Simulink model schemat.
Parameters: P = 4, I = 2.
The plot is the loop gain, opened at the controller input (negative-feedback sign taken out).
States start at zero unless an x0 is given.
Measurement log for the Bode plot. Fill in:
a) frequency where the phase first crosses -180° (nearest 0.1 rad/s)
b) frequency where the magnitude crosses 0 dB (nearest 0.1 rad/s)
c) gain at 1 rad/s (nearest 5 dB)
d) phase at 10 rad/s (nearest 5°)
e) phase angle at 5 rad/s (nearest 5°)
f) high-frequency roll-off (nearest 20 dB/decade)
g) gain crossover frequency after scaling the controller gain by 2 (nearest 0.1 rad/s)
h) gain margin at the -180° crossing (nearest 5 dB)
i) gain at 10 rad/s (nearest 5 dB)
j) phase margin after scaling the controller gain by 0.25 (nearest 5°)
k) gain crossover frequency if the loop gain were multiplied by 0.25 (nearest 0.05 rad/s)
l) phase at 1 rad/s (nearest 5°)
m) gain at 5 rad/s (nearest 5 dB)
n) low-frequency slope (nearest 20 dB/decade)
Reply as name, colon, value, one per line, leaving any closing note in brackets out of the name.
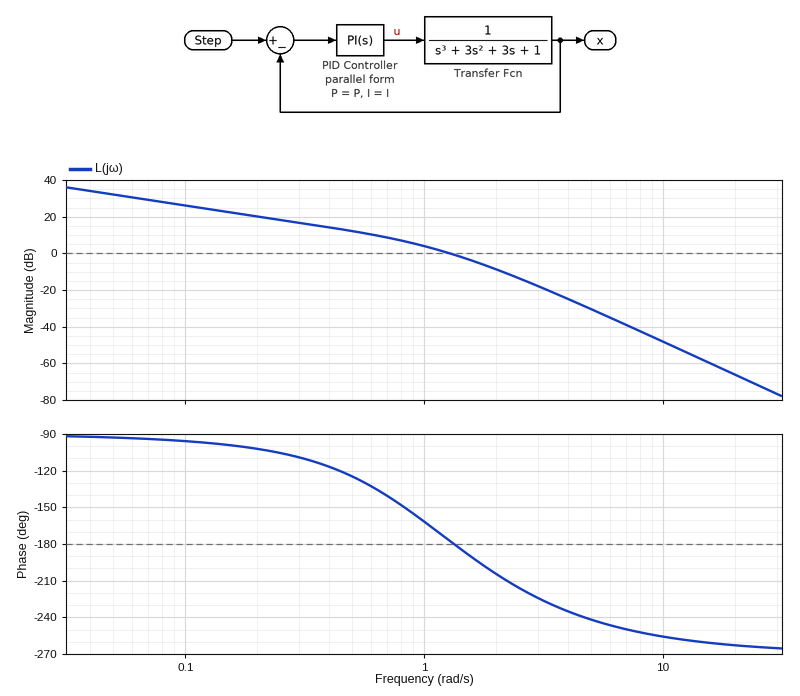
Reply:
frequency where the phase first crosses -180°: 1.3 rad/s
frequency where the magnitude crosses 0 dB: 1.3 rad/s
gain at 1 rad/s: 5 dB
phase at 10 rad/s: -255°
phase angle at 5 rad/s: -240°
high-frequency roll-off: -60 dB/decade
gain crossover frequency after scaling the controller gain by 2: 1.8 rad/s
gain margin at the -180° crossing: 0 dB
gain at 10 rad/s: -50 dB
phase margin after scaling the controller gain by 0.25: 55°
gain crossover frequency if the loop gain were multiplied by 0.25: 0.50 rad/s
phase at 1 rad/s: -160°
gain at 5 rad/s: -30 dB
low-frequency slope: -20 dB/decade
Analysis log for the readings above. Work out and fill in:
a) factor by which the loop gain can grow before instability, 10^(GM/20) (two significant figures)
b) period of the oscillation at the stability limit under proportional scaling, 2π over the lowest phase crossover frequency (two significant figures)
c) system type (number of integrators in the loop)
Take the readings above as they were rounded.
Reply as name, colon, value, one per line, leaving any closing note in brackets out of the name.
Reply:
factor by which the loop gain can grow before instability, 10^(GM/20): 1.0
period of the oscillation at the stability limit under proportional scaling, 2π over the lowest phase crossover frequency: 4.8 s
system type: 1
